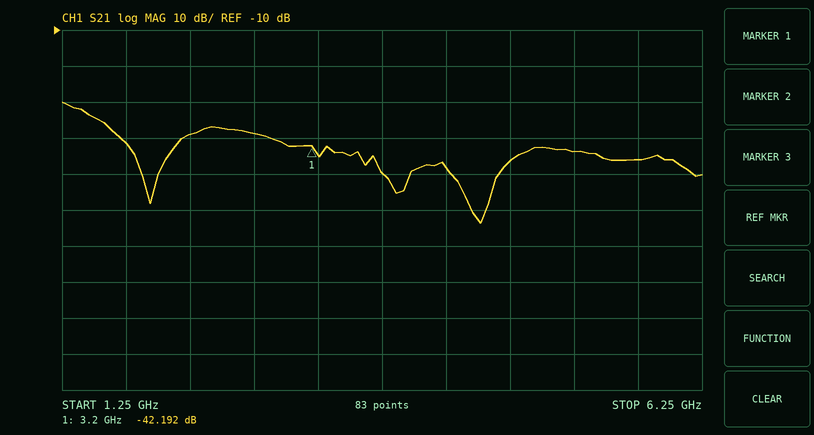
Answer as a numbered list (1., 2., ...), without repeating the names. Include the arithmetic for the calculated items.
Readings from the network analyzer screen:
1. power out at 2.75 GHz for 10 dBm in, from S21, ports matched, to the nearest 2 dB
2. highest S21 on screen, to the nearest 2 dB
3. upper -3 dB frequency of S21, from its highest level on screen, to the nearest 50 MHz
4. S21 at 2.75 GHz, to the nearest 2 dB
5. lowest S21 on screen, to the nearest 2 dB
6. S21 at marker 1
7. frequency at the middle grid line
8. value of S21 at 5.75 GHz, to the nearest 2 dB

1. 10 dBm + (-38 dB) = -28 dBm
2. -30 dB
3. 1.45 GHz
4. -38 dB
5. -64 dB
6. -42.192 dB
7. 3.75 GHz
8. -46 dB
